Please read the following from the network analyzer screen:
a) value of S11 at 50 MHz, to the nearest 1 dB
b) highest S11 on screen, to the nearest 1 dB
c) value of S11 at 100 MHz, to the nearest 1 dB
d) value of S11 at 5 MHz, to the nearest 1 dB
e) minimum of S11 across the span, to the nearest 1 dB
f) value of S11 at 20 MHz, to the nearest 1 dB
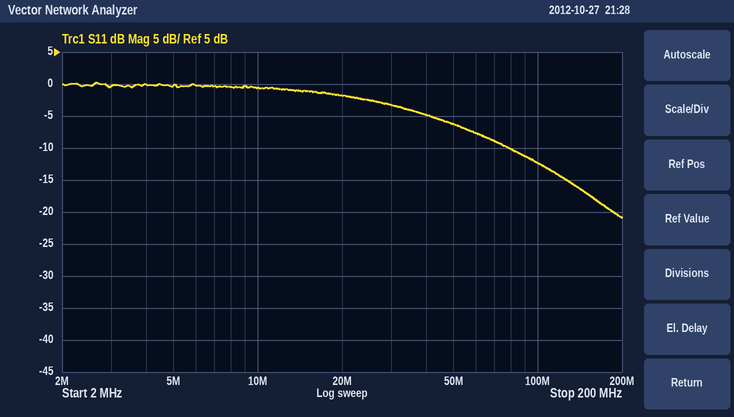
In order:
-6 dB
0 dB
-12 dB
0 dB
-21 dB
-2 dB
